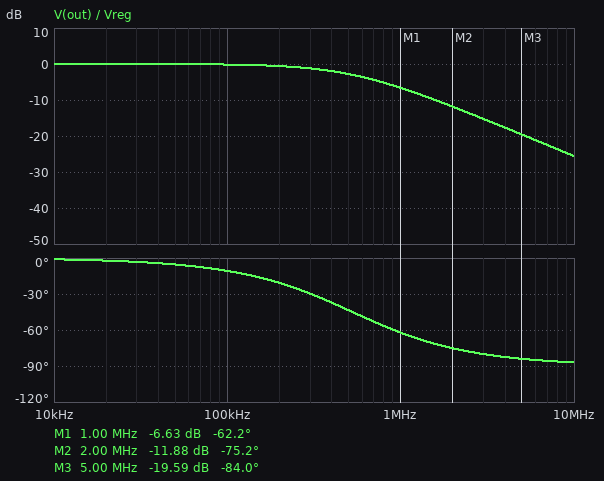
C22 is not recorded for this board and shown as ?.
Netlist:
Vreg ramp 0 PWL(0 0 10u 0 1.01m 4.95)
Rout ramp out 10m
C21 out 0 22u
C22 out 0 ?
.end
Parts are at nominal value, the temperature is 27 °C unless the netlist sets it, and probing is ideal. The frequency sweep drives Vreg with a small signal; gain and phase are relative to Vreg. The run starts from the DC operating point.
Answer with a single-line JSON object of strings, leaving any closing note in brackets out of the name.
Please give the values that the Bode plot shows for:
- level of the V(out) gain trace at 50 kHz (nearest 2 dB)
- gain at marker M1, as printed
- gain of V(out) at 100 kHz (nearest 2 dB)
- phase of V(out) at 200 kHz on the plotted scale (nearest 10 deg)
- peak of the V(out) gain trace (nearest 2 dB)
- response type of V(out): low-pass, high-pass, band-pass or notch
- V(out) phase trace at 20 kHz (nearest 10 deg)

{"level of the V(out) gain trace at 50 kHz": "0 dB", "gain at marker M1, as printed": "-6.63 dB", "gain of V(out) at 100 kHz": "0 dB", "phase of V(out) at 200 kHz on the plotted scale": "-20 deg", "peak of the V(out) gain trace": "0 dB", "response type of V(out): low-pass, high-pass, band-pass or notch": "low-pass", "V(out) phase trace at 20 kHz": "0 deg"}
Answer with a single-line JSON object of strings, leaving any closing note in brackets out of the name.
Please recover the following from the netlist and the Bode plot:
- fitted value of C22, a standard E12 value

{"fitted value of C22, a standard E12 value": "8.2 µF"}
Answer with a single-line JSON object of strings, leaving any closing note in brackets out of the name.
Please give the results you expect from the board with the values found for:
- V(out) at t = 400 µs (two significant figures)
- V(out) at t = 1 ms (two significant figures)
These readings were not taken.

{"V(out) at t = 400 µs": "1.9 V", "V(out) at t = 1 ms": "4.9 V"}
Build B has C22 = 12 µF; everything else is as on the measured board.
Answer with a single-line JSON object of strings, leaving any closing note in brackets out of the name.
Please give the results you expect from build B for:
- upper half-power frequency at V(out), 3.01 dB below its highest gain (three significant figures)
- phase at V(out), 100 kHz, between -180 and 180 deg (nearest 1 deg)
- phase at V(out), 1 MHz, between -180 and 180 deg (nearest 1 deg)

{"upper half-power frequency at V(out), 3.01 dB below its highest gain": "468 kHz", "phase at V(out), 100 kHz, between -180 and 180 deg": "-12 deg", "phase at V(out), 1 MHz, between -180 and 180 deg": "-65 deg"}
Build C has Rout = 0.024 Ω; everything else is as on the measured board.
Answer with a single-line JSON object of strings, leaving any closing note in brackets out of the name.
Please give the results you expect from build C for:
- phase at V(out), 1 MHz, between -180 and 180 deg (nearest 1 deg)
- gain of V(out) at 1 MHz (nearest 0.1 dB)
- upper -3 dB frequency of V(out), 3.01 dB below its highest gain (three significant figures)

{"phase at V(out), 1 MHz, between -180 and 180 deg": "-78 deg", "gain of V(out) at 1 MHz": "-13.4 dB", "upper -3 dB frequency of V(out), 3.01 dB below its highest gain": "220 kHz"}
